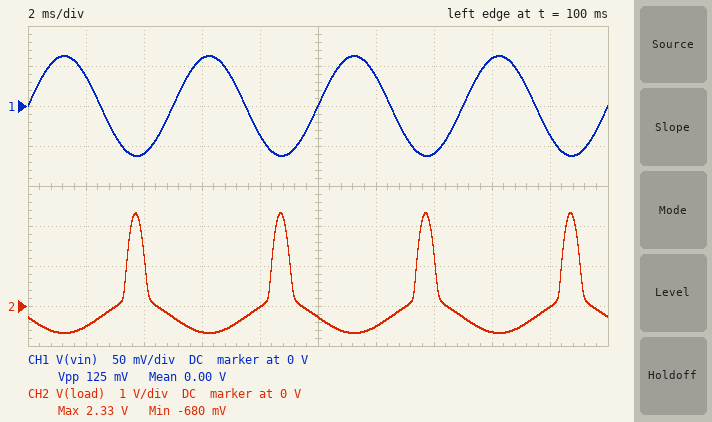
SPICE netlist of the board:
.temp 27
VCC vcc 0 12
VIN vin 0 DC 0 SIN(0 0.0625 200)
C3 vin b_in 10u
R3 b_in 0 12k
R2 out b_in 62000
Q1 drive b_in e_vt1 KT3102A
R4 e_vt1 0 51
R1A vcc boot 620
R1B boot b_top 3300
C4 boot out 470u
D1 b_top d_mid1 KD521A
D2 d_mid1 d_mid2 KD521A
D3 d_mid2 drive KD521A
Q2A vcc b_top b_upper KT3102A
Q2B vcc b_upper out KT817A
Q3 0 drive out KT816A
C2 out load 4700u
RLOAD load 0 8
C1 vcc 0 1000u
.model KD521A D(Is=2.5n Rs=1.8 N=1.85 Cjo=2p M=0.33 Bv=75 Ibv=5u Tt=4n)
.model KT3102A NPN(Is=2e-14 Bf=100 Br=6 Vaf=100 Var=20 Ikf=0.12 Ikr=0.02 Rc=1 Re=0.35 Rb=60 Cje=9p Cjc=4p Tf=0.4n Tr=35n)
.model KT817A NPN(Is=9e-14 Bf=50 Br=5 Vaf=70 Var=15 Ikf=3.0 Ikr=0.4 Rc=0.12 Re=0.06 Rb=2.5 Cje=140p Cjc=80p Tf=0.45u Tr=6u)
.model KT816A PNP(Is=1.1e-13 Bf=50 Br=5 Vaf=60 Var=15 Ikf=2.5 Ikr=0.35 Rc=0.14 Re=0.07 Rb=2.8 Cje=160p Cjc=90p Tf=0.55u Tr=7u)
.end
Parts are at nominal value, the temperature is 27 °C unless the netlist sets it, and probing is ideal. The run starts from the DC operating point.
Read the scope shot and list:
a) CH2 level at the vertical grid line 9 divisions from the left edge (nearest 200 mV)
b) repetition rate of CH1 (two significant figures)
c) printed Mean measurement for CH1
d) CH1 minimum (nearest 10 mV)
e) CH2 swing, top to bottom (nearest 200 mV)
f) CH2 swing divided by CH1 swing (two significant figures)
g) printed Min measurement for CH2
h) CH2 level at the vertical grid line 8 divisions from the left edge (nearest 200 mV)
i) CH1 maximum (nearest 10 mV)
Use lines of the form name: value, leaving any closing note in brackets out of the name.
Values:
CH2 level at the vertical grid line 9 divisions from the left edge: 0 V
repetition rate of CH1: 200 Hz
printed Mean measurement for CH1: 0.00 V
CH1 minimum: -60 mV
CH2 swing, top to bottom: 3.0 V
CH2 swing divided by CH1 swing: 24
printed Min measurement for CH2: -680 mV
CH2 level at the vertical grid line 8 divisions from the left edge: -600 mV
CH1 maximum: 60 mV
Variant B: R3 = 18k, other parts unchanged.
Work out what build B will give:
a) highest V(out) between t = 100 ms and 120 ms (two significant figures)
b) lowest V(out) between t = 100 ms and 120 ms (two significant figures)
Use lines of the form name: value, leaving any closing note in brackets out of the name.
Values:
highest V(out) between t = 100 ms and 120 ms: 7.3 V
lowest V(out) between t = 100 ms and 120 ms: 4.3 V
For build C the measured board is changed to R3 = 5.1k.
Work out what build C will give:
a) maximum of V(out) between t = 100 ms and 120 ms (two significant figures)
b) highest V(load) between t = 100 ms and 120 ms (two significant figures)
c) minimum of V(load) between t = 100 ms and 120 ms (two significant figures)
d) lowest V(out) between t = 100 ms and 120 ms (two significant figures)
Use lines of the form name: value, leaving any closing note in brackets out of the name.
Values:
maximum of V(out) between t = 100 ms and 120 ms: 11 V
highest V(load) between t = 100 ms and 120 ms: 1.6 V
minimum of V(load) between t = 100 ms and 120 ms: -560 mV
lowest V(out) between t = 100 ms and 120 ms: 9.0 V
